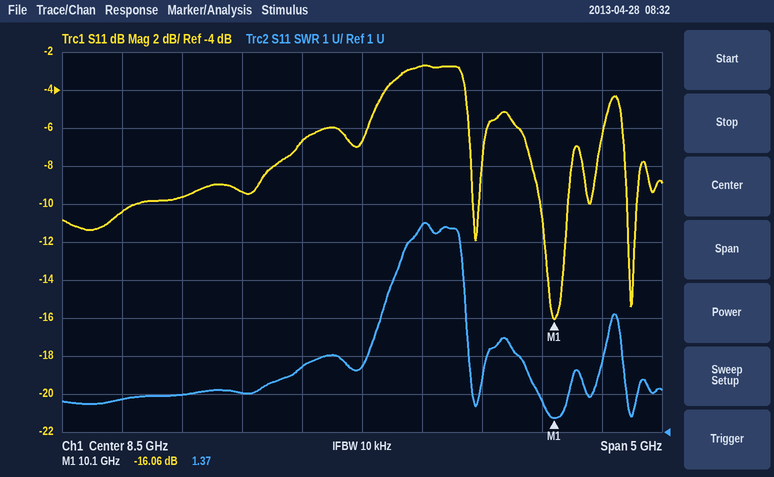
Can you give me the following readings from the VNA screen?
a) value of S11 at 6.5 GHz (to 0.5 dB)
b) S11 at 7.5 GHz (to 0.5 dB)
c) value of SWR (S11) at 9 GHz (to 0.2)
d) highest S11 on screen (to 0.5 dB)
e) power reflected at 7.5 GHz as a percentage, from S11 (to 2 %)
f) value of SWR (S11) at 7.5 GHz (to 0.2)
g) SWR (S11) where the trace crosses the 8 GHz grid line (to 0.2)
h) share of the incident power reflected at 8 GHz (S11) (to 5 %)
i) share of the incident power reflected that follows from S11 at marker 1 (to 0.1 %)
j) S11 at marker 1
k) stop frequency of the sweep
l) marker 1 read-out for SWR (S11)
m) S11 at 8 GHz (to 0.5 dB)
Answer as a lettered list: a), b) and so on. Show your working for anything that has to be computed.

a) -10.5 dB
b) -9.5 dB
c) 6.4
d) -2.5 dB
e) 10^(-9.5/10) ≈ 11.2 %, so 12 % to the nearest 2 %
f) 2.0
g) 2.8
h) 10^(-6.5/10) ≈ 22.4 %, so 20 % to the nearest 5 %
i) 10^(-16.06/10) ≈ 2.5 %
j) -16.06 dB
k) 11 GHz
l) 1.37
m) -6.5 dB
